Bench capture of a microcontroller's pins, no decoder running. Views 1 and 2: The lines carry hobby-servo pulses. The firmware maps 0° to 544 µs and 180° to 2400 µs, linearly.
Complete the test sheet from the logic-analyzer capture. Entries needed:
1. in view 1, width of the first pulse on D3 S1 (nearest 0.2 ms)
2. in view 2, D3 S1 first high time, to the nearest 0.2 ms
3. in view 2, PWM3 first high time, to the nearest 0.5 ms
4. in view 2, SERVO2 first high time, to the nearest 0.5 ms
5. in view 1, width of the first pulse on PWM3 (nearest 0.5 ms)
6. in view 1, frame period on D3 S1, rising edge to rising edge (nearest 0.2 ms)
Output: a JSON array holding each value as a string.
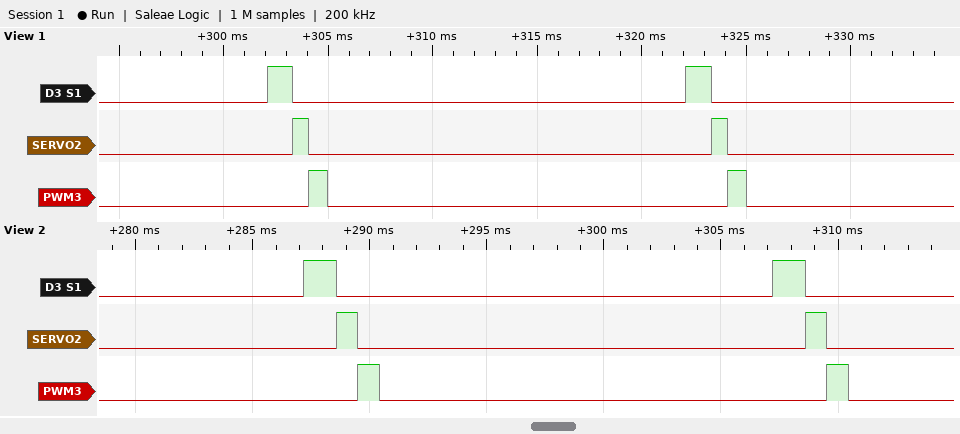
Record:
["1.2 ms", "1.4 ms", "1.0 ms", "1.0 ms", "1.0 ms", "20.0 ms"]
